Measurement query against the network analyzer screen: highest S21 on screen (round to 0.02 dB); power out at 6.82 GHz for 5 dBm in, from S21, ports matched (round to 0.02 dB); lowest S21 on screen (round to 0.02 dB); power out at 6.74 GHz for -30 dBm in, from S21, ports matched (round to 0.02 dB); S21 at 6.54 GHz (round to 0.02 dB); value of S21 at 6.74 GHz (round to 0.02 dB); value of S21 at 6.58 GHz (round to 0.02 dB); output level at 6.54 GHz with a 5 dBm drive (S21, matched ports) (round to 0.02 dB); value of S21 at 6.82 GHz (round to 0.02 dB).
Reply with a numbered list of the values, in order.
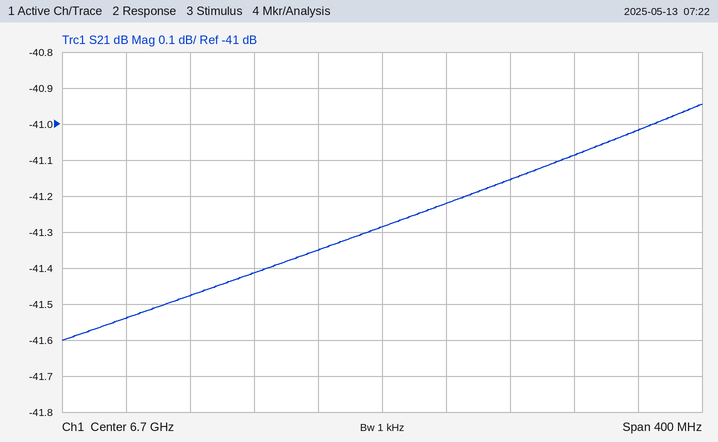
1. -40.94 dB
2. -36.08 dBm
3. -41.60 dB
4. -71.22 dBm
5. -41.54 dB
6. -41.22 dB
7. -41.48 dB
8. -36.54 dBm
9. -41.08 dB
